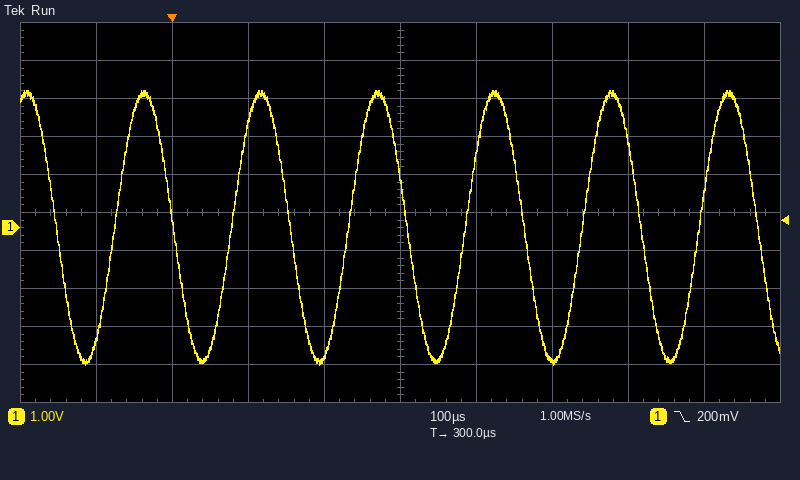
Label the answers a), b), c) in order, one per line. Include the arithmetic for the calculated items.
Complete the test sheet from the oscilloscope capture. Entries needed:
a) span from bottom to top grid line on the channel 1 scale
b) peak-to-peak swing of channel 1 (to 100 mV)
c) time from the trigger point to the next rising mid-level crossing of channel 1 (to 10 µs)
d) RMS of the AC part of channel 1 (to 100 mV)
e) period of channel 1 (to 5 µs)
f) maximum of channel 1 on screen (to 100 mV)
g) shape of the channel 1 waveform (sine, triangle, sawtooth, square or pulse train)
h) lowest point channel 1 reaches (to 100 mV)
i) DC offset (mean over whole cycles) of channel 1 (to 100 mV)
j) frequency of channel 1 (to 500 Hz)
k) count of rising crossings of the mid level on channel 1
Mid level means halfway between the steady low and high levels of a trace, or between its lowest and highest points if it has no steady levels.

a) 10 V
b) 3.6 V − (-3.6 V) = 7.2 V
c) 80 µs
d) 7.2 V / (2√2) ≈ 2.5 V
e) 155 µs
f) 3.6 V
g) sine
h) -3.6 V
i) (3.6 V + (-3.6 V)) / 2 ≈ 0.0 V
j) 1 / 155 µs ≈ 6.5 kHz
k) 6
